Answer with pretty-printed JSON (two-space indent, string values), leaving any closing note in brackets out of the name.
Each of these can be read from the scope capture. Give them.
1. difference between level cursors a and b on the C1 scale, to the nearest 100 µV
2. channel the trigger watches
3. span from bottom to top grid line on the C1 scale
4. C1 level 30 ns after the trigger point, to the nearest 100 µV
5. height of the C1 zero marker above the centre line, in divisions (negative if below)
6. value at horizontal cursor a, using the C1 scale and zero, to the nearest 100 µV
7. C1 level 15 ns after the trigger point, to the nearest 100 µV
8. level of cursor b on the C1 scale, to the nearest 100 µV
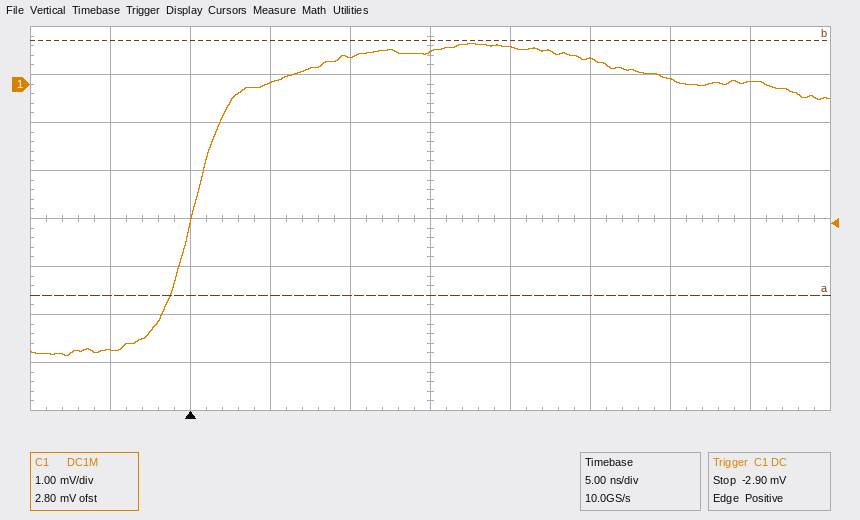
{
  "difference between level cursors a and b on the C1 scale, to the nearest 100 µV": "5.3 mV",
  "channel the trigger watches": "C1",
  "span from bottom to top grid line on the C1 scale": "8 mV",
  "C1 level 30 ns after the trigger point, to the nearest 100 µV": "100 µV",
  "height of the C1 zero marker above the centre line, in divisions": "+2.8 div",
  "value at horizontal cursor a, using the C1 scale and zero, to the nearest 100 µV": "-4.4 mV",
  "C1 level 15 ns after the trigger point, to the nearest 100 µV": "700 µV",
  "level of cursor b on the C1 scale, to the nearest 100 µV": "900 µV"
}
